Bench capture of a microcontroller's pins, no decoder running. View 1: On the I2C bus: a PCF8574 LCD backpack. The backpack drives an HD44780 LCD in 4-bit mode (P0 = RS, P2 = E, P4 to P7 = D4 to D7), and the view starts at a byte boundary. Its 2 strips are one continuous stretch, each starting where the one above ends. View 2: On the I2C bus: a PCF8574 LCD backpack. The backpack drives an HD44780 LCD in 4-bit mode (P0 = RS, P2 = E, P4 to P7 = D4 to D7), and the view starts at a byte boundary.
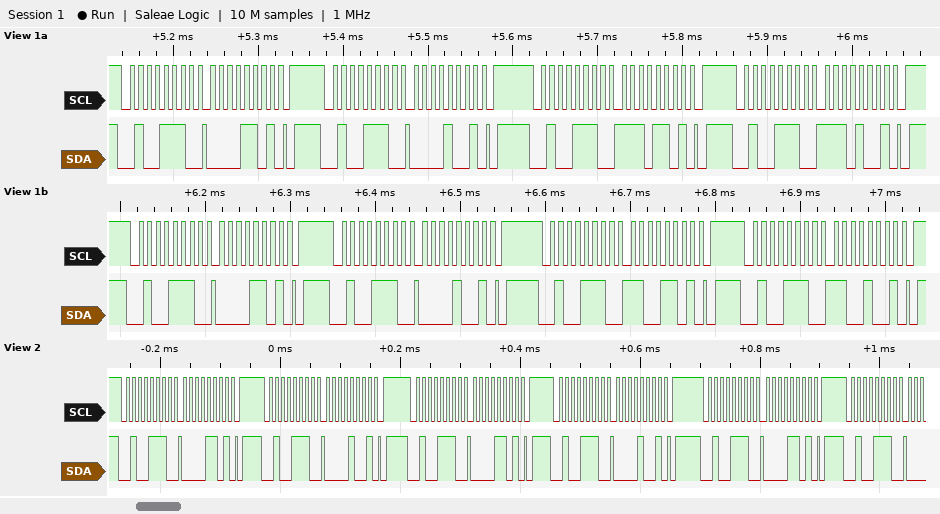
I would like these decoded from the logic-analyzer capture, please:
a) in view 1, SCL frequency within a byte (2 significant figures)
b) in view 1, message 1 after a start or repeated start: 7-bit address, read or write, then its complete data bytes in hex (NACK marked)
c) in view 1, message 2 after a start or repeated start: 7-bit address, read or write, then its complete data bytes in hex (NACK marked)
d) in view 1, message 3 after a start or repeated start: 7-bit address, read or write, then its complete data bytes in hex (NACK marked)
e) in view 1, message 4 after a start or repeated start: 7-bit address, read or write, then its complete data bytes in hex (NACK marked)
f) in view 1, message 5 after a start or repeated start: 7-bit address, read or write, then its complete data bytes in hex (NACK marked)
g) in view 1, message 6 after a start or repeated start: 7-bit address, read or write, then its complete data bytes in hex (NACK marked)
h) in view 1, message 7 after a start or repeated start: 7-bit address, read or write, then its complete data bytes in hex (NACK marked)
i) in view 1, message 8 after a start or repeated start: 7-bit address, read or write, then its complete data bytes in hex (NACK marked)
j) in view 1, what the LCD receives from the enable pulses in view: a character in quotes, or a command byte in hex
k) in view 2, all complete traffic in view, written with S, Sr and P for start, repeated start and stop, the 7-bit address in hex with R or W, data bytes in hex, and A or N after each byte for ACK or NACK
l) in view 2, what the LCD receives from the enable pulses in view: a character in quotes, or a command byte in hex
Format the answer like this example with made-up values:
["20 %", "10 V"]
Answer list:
["100 kHz", "0x27 write: 0D", "0x27 write: 09", "0x27 write: ED", "0x27 write: E9", "0x27 write: 0D", "0x27 write: 09", "0x27 write: CD", "0x27 write: C9", "data 0x0E data 0x0C", "S 27W A 0D A P S 27W A 09 A P S 27W A 0D A P S 27W A 09 A P S 27W A 0D A P S 27W A", "data 0x00"]
